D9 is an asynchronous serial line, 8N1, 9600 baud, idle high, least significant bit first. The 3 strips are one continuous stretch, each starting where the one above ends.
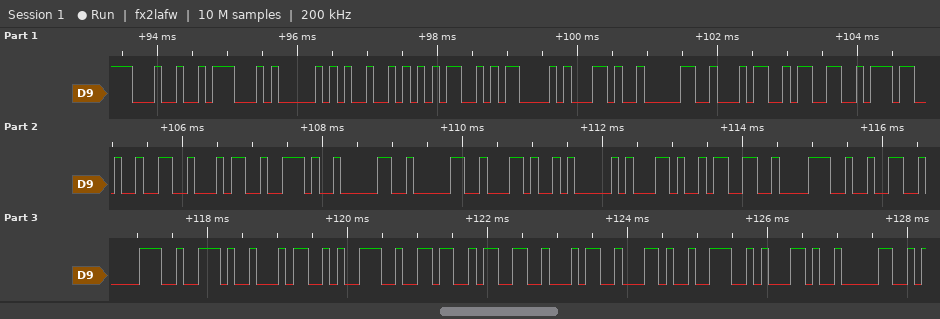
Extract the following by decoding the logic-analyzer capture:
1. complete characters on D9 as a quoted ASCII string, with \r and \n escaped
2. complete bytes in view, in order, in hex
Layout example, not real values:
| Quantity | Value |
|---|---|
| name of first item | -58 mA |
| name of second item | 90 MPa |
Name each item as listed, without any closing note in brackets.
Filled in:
| Quantity | Value |
|---|---|
| complete characters on D9 as a quoted ASCII string, with \r and \n escaped | "$GPRMC,043724.00,A,3828.49634,N,0" |
| complete bytes in view, in order, in hex | 24 47 50 52 4D 43 2C 30 34 33 37 32 34 2E 30 30 2C 41 2C 33 38 32 38 2E 34 39 36 33 34 2C 4E 2C 30 |
